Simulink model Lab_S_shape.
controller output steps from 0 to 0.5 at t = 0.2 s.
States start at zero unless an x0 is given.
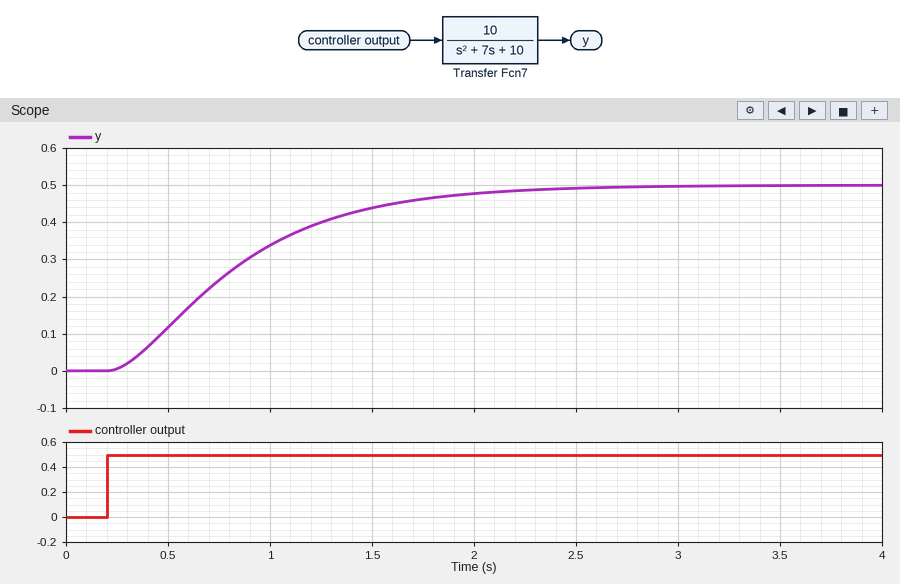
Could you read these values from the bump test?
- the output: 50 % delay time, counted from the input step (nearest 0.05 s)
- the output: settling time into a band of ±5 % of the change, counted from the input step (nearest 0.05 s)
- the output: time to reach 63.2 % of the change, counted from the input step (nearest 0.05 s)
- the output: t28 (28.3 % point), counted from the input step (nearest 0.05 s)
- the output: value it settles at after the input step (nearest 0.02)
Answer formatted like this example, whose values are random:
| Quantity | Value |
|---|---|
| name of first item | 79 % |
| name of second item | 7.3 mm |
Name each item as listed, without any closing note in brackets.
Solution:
| Quantity | Value |
|---|---|
| the output: 50 % delay time, counted from the input step | 0.55 s |
| the output: settling time into a band of ±5 % of the change, counted from the input step | 1.75 s |
| the output: time to reach 63.2 % of the change, counted from the input step | 0.75 s |
| the output: t28 (28.3 % point), counted from the input step | 0.35 s |
| the output: value it settles at after the input step | 0.50 |
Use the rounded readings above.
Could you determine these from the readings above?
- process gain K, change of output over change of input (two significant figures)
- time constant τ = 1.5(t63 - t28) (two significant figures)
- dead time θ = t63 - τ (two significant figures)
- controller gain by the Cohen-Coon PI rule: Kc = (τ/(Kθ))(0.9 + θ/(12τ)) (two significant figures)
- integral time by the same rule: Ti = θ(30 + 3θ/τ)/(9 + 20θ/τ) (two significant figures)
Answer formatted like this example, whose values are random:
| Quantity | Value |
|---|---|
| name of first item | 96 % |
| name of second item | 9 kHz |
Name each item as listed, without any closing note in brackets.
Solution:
| Quantity | Value |
|---|---|
| process gain K, change of output over change of input | 1.0 |
| time constant τ = 1.5(t63 - t28) | 0.60 s |
| dead time θ = t63 - τ | 0.15 s |
| controller gain by the Cohen-Coon PI rule: Kc = (τ/(Kθ))(0.9 + θ/(12τ)) | 3.7 |
| integral time by the same rule: Ti = θ(30 + 3θ/τ)/(9 + 20θ/τ) | 0.33 s |
